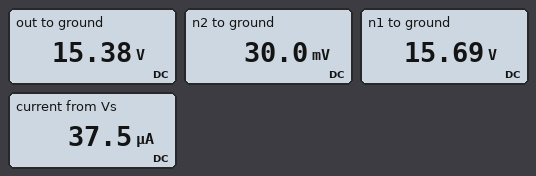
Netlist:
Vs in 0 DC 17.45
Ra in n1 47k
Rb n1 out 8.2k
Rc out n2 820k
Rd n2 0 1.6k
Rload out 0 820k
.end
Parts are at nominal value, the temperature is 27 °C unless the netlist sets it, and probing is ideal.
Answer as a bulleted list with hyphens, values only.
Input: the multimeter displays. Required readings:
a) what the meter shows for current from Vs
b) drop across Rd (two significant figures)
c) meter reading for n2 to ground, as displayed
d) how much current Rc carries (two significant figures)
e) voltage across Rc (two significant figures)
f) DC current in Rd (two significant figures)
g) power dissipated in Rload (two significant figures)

- 37.5 µA
- 30 mV
- 30.0 mV
- 19 µA
- 15 V
- 19 µA
- 290 µW
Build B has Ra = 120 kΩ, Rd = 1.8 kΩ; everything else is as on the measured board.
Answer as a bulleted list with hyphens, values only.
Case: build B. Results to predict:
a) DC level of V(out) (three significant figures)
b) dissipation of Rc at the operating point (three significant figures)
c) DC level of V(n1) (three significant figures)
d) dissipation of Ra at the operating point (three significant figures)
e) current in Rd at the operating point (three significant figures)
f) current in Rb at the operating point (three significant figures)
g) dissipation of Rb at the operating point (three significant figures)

- 13.3 V
- 215 µW
- 13.6 V
- 126 µW
- 16.2 µA
- 32.4 µA
- 8.61 µW
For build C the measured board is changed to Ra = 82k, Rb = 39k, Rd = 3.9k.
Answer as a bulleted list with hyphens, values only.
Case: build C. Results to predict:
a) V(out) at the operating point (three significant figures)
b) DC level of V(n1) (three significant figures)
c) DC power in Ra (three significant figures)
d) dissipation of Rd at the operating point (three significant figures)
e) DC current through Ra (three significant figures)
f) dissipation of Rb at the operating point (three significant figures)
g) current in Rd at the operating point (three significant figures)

- 13.5 V
- 14.8 V
- 88.2 µW
- 1.04 µW
- 32.8 µA
- 42.0 µW
- 16.4 µA
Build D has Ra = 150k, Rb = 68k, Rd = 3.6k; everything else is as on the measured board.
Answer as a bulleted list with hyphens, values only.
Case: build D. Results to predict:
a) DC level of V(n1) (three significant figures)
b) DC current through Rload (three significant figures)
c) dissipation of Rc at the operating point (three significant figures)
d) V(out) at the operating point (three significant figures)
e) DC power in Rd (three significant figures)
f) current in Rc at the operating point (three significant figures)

- 13.3 V
- 13.9 µA
- 157 µW
- 11.4 V
- 690 nW
- 13.8 µA
